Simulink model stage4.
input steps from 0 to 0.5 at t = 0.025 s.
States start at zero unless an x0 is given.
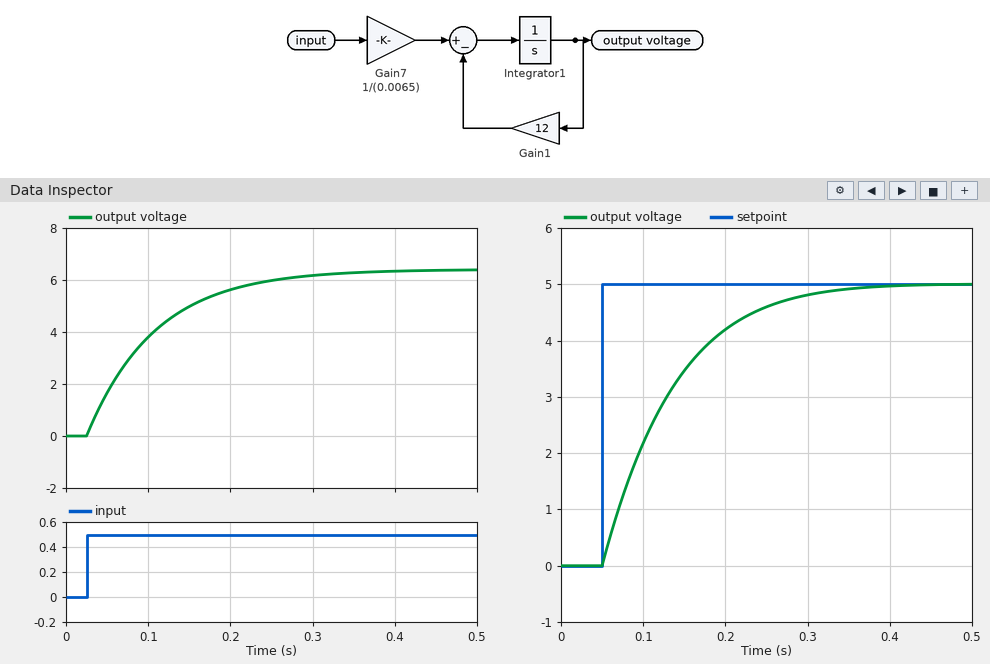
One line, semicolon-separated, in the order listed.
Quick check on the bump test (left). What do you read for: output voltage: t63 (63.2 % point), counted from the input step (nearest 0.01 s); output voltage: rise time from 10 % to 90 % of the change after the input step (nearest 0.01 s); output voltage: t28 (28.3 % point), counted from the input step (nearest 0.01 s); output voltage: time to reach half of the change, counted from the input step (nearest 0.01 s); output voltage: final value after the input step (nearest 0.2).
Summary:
0.08 s; 0.18 s; 0.03 s; 0.06 s; 6.4
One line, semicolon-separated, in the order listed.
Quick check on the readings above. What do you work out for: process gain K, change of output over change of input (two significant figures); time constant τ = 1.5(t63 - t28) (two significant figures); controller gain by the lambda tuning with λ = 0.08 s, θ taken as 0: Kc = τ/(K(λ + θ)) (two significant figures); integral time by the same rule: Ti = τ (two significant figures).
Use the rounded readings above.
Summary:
13; 0.075 s; 0.072; 0.075 s
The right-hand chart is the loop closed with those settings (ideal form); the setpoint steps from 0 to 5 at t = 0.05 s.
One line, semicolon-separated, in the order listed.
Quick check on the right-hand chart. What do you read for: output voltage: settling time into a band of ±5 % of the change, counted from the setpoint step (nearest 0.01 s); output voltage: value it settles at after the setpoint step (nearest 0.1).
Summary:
0.23 s; 5.0
